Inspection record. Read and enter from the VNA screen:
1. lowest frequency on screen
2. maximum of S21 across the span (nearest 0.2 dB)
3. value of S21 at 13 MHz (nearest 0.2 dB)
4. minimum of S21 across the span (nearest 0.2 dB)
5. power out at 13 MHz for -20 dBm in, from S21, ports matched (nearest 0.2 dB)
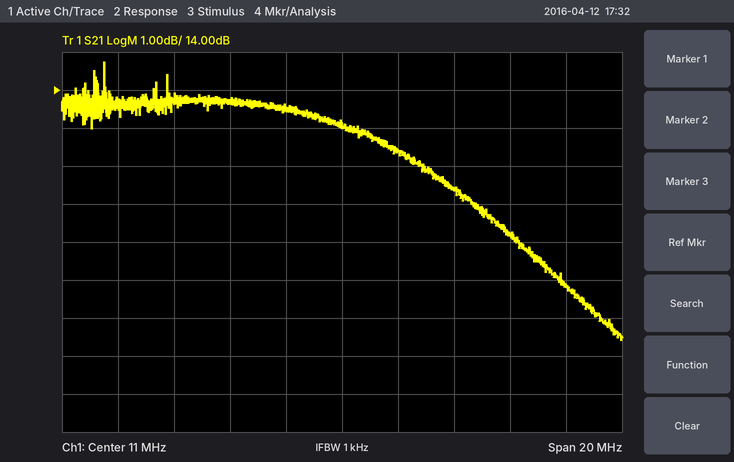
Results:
1 MHz
14.8 dB
12.4 dB
7.4 dB
-7.6 dBm
